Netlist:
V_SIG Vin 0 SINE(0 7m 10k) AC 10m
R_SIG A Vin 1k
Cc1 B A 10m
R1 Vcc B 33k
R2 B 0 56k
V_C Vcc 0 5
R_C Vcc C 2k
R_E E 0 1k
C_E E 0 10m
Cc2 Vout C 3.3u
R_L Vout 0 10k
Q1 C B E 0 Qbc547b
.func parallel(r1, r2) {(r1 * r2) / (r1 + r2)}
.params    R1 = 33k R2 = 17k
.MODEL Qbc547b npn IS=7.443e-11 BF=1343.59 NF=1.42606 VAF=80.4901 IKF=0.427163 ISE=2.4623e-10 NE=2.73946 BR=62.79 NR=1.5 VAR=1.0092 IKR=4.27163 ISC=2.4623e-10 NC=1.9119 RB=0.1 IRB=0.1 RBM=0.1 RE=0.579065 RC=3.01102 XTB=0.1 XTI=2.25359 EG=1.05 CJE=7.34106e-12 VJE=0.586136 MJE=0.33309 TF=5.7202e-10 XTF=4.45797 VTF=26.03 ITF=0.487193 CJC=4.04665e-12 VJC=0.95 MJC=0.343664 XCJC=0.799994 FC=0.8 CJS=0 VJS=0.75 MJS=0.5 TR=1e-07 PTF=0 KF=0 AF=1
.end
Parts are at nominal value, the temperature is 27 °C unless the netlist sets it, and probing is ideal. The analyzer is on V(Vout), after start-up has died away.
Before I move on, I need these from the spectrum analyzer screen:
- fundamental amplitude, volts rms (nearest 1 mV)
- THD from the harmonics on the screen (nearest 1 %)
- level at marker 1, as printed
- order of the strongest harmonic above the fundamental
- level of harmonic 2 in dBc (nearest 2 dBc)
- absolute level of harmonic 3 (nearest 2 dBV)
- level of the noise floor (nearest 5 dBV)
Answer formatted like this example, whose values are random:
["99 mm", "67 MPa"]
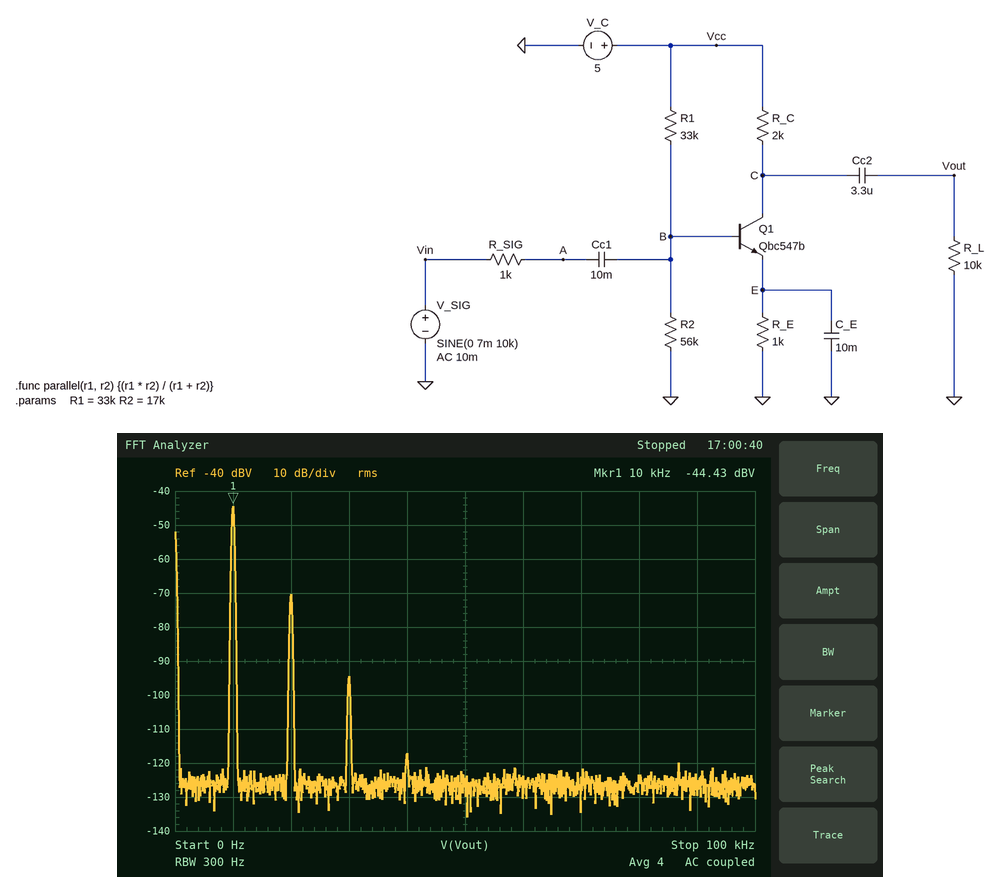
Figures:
["6 mV", "5 %", "-44.43 dBV", "2", "-26 dBc", "-94 dBV", "-125 dBV"]
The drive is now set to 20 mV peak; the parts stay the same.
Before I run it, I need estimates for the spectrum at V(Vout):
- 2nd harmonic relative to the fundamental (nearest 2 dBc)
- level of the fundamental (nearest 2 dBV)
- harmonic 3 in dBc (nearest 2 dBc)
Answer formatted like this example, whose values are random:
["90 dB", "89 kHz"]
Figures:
["-16 dBc", "-34 dBV", "-30 dBc"]
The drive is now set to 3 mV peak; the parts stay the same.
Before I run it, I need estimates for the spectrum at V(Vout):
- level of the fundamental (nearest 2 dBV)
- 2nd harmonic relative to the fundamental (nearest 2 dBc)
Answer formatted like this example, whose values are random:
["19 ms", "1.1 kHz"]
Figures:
["-52 dBV", "-34 dBc"]
